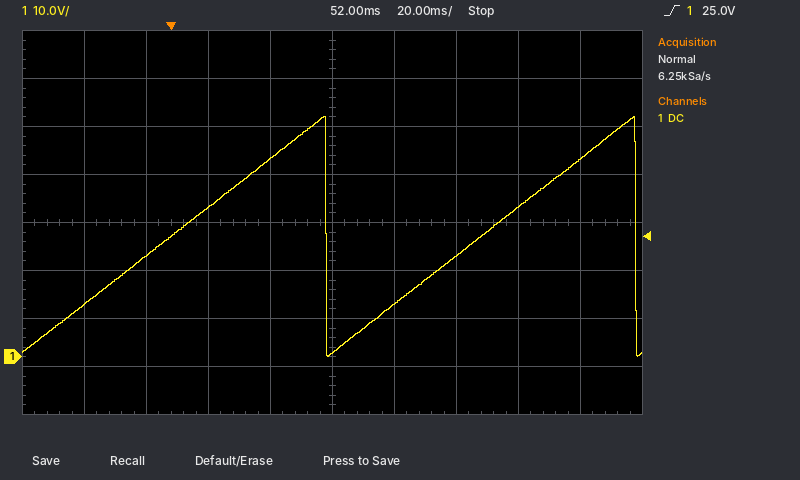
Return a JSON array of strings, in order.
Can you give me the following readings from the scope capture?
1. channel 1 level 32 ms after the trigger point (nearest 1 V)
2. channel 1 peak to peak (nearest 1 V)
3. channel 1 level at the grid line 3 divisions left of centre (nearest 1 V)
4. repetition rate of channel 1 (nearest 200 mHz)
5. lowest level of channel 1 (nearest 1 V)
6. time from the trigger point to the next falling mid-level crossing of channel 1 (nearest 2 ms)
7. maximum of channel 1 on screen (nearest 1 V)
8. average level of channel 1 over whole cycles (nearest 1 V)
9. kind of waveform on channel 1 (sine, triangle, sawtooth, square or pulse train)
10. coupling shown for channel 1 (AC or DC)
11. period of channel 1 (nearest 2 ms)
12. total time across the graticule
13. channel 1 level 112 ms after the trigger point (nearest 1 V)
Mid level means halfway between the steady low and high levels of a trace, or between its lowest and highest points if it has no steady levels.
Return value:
["41 V", "50 V", "21 V", "10.0 Hz", "0 V", "50 ms", "50 V", "25 V", "sawtooth", "DC", "100 ms", "200 ms", "31 V"]
